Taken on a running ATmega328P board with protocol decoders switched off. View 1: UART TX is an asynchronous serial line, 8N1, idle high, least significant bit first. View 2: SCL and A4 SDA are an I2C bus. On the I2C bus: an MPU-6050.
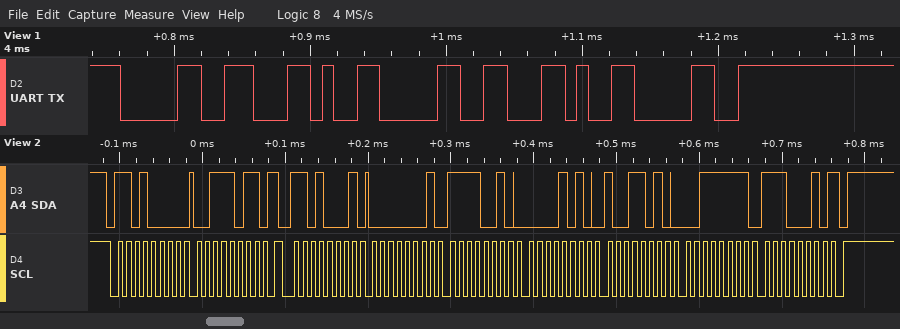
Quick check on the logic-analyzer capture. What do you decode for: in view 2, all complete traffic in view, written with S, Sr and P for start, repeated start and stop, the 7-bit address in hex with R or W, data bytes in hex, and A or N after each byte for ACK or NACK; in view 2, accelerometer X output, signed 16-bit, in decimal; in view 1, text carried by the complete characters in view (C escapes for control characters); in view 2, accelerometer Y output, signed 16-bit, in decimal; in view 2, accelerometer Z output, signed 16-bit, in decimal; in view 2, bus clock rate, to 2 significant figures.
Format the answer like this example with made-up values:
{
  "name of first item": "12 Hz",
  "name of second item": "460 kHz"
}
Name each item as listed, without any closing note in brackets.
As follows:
{
  "in view 2, all complete traffic in view, written with S, Sr and P for start, repeated start and stop, the 7-bit address in hex with R or W, data bytes in hex, and A or N after each byte for ACK or NACK": "S 68W A 3B A Sr 68R A 01 A F2 A 0A A 9A A 3F A E2 N P",
  "in view 2, accelerometer X output, signed 16-bit, in decimal": "498",
  "in view 1, text carried by the complete characters in view": "\"0,0,0\"",
  "in view 2, accelerometer Y output, signed 16-bit, in decimal": "2714",
  "in view 2, accelerometer Z output, signed 16-bit, in decimal": "16354",
  "in view 2, bus clock rate, to 2 significant figures": "100 kHz"
}
